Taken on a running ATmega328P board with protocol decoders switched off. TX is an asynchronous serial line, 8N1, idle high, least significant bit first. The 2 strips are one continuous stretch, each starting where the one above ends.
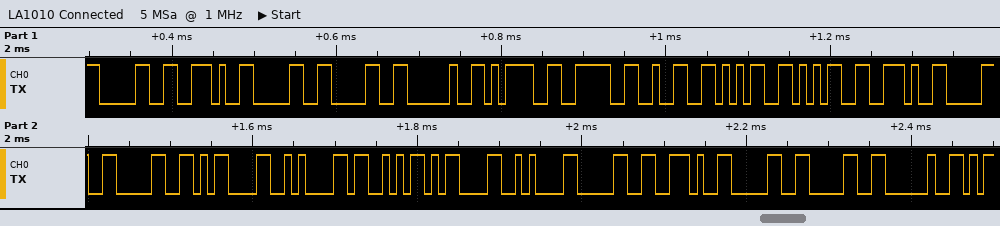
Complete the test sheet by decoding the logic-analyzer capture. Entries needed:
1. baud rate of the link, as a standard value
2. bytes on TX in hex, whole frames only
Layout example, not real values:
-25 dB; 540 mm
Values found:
115200 baud; 0x30 0x2E 0x30 0x30 0x20 0x3D 0x3E 0x32 0x35 0x35 0x2E 0x30 0x30 0x0D 0x0A 0x53 0x0D 0x0A 0x30 0x2E 0x30 0x30 0x20
